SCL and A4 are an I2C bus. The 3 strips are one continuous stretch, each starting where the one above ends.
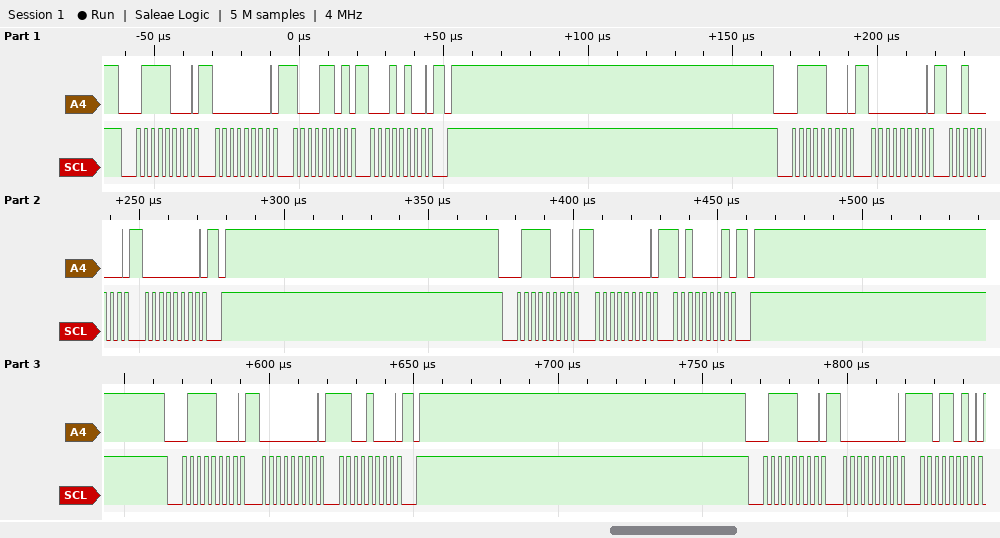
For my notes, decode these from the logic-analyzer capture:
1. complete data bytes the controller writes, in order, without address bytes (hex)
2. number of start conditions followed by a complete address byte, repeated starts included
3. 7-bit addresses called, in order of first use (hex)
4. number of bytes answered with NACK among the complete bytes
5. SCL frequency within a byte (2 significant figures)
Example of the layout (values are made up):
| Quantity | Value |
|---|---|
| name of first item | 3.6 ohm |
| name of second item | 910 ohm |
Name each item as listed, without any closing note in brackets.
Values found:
| Quantity | Value |
|---|---|
| complete data bytes the controller writes, in order, without address bytes | 00 8D 14 00 20 00 00 A1 00 C8 00 DA |
| number of start conditions followed by a complete address byte, repeated starts included | 5 |
| 7-bit addresses called, in order of first use | 0x3C |
| number of bytes answered with NACK among the complete bytes | 0 |
| SCL frequency within a byte | 400 kHz |
